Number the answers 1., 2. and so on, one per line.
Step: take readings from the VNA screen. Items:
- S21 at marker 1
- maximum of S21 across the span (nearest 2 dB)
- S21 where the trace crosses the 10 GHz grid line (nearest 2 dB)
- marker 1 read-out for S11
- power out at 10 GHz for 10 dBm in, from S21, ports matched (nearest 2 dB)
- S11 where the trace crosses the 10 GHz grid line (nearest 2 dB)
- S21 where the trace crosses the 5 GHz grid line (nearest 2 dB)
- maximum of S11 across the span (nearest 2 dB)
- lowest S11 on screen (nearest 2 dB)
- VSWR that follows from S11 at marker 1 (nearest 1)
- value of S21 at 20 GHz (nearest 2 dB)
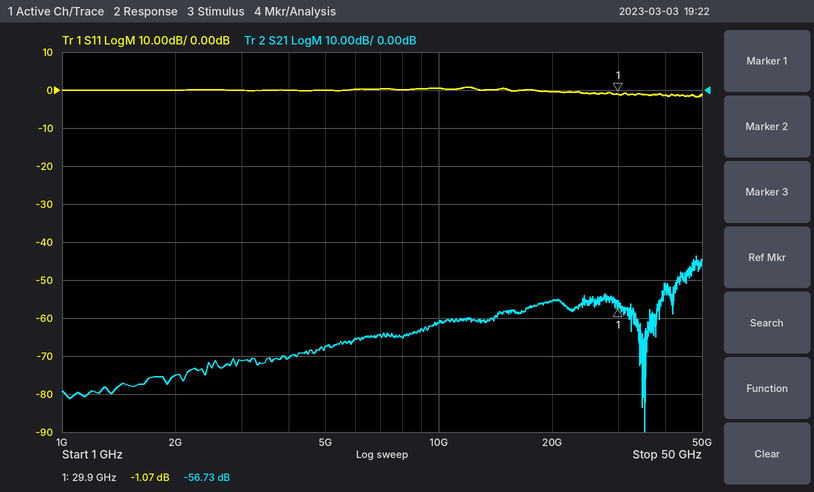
1. -56.73 dB
2. -44 dB
3. -62 dB
4. -1.07 dB
5. -52 dBm
6. 0 dB
7. -68 dB
8. 0 dB
9. -2 dB
10. 16
11. -56 dB
